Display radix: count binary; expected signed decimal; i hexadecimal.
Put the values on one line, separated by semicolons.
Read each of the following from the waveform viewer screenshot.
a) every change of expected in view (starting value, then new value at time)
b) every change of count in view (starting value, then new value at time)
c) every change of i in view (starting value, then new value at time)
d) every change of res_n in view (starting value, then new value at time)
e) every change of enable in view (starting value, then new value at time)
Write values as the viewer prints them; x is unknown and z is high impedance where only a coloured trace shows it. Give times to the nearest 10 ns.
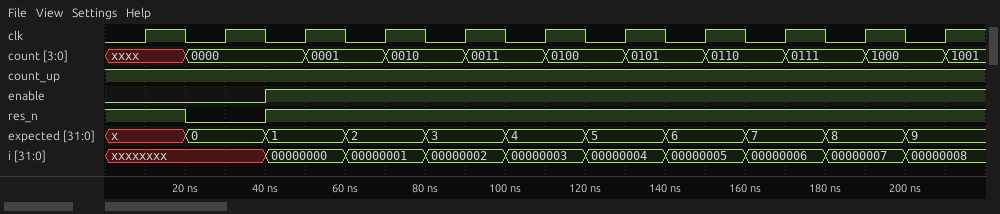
x, 0 at 20 ns, 1 at 40 ns, 2 at 60 ns, 3 at 80 ns, 4 at 100 ns, 5 at 120 ns, 6 at 140 ns, 7 at 160 ns, 8 at 180 ns, 9 at 200 ns; xxxx, 0000 at 20 ns, 0001 at 50 ns, 0010 at 70 ns, 0011 at 90 ns, 0100 at 110 ns, 0101 at 130 ns, 0110 at 150 ns, 0111 at 170 ns, 1000 at 190 ns, 1001 at 210 ns; xxxxxxxx, 00000000 at 40 ns, 00000001 at 60 ns, 00000002 at 80 ns, 00000003 at 100 ns, 00000004 at 120 ns, 00000005 at 140 ns, 00000006 at 160 ns, 00000007 at 180 ns, 00000008 at 200 ns; 1, 0 at 20 ns, 1 at 40 ns; 0, 1 at 40 ns
